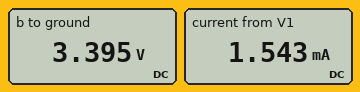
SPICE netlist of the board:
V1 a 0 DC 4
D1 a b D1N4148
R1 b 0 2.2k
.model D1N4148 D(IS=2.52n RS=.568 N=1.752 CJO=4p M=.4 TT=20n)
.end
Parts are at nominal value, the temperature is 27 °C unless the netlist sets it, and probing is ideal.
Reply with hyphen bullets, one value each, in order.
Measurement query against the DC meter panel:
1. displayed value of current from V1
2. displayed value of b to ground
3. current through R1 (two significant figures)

- 1.543 mA
- 3.395 V
- 1.5 mA
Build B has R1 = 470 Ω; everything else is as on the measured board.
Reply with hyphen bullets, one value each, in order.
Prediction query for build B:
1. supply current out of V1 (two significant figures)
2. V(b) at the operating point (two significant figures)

- 7.1 mA
- 3.3 V
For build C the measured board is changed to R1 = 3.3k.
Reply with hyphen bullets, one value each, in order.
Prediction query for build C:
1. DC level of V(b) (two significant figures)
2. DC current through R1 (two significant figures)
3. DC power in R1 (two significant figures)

- 3.4 V
- 1.0 mA
- 3.5 mW
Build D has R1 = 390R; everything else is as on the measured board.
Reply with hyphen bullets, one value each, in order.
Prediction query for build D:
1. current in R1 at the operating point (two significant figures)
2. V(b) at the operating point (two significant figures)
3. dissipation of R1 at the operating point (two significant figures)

- 8.5 mA
- 3.3 V
- 28 mW
